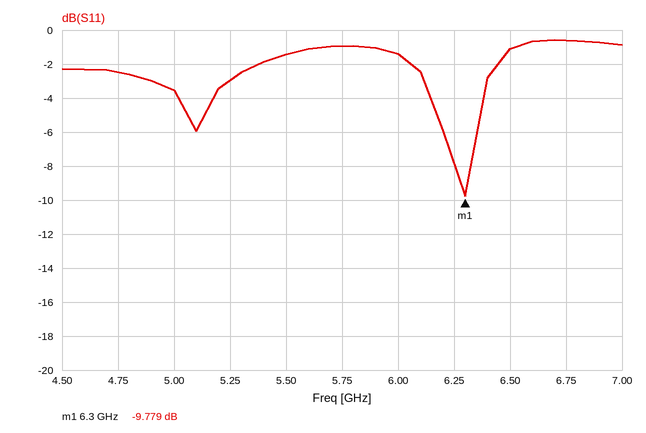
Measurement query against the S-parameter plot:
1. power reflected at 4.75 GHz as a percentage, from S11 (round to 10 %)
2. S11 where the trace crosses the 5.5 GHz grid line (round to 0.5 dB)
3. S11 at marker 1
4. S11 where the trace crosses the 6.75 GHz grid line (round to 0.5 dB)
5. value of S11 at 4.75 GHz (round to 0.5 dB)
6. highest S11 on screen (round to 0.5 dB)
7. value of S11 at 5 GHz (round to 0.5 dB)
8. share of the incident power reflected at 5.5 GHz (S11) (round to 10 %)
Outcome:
60 %
-1.5 dB
-9.779 dB
-0.5 dB
-2.5 dB
-0.5 dB
-3.5 dB
70 %
